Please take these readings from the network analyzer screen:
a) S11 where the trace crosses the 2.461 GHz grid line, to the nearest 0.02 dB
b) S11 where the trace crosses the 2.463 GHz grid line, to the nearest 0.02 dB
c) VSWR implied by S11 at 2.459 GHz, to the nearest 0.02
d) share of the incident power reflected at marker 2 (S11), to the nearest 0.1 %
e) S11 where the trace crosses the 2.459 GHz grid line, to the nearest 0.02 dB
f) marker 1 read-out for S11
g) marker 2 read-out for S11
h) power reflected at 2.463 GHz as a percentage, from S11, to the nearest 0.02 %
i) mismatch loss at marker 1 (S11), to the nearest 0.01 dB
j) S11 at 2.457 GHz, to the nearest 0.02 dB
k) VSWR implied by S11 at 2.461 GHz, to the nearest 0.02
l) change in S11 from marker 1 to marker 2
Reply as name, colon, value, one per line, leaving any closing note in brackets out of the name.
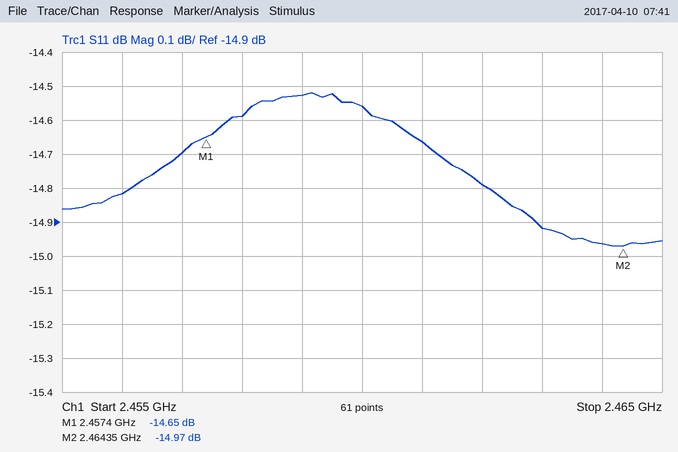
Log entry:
S11 where the trace crosses the 2.461 GHz grid line, to the nearest 0.02 dB: -14.66 dB
S11 where the trace crosses the 2.463 GHz grid line, to the nearest 0.02 dB: -14.92 dB
VSWR implied by S11 at 2.459 GHz, to the nearest 0.02: 1.46
share of the incident power reflected at marker 2 (S11), to the nearest 0.1 %: 3.2 %
S11 where the trace crosses the 2.459 GHz grid line, to the nearest 0.02 dB: -14.52 dB
marker 1 read-out for S11: -14.65 dB
marker 2 read-out for S11: -14.97 dB
power reflected at 2.463 GHz as a percentage, from S11, to the nearest 0.02 %: 3.22 %
mismatch loss at marker 1 (S11), to the nearest 0.01 dB: 0.15 dB
S11 at 2.457 GHz, to the nearest 0.02 dB: -14.70 dB
VSWR implied by S11 at 2.461 GHz, to the nearest 0.02: 1.46
change in S11 from marker 1 to marker 2: -0.32 dB
